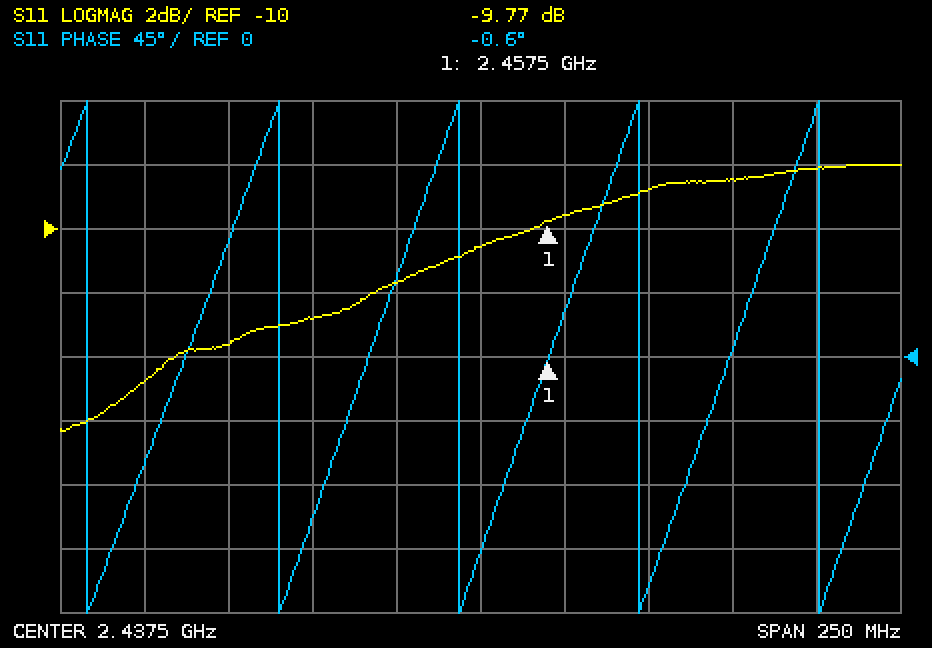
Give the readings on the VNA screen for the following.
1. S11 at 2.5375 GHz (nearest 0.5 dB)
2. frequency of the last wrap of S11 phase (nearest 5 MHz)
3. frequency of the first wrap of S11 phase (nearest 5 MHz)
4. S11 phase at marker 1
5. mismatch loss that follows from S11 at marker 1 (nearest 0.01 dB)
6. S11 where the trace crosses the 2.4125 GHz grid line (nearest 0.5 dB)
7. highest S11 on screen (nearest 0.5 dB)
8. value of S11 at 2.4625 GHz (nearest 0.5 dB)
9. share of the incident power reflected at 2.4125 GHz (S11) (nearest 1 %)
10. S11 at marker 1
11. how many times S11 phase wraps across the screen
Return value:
-8.0 dB
2.540 GHz
2.320 GHz
-0.6°
0.48 dB
-11.5 dB
-8.0 dB
-9.5 dB
7 %
-9.77 dB
5
